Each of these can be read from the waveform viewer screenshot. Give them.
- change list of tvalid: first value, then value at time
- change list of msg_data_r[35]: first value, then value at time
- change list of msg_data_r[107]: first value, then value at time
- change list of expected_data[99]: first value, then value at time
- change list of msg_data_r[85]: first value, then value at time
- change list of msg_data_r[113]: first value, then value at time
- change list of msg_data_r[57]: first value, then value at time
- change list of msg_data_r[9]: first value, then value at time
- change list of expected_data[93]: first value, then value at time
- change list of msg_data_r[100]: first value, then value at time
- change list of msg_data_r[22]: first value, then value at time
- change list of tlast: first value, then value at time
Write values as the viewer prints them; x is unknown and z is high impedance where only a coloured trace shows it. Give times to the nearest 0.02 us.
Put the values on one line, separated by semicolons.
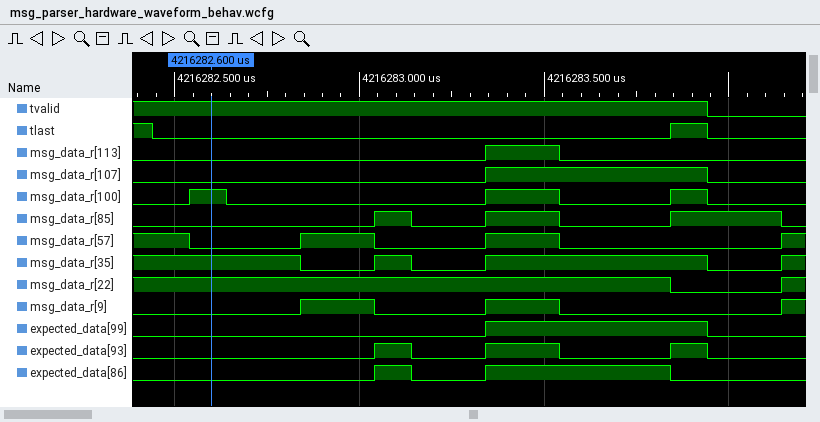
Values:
1, 0 at 4216283.94 us; 1, 0 at 4216282.84 us, 1 at 4216283.04 us, 0 at 4216283.14 us, 1 at 4216283.34 us, 0 at 4216283.94 us, 1 at 4216284.14 us; 0, 1 at 4216283.34 us, 0 at 4216283.94 us; 0, 1 at 4216283.34 us, 0 at 4216283.94 us; 0, 1 at 4216283.04 us, 0 at 4216283.14 us, 1 at 4216283.34 us, 0 at 4216283.54 us, 1 at 4216283.84 us, 0 at 4216284.14 us; 0, 1 at 4216283.34 us, 0 at 4216283.54 us; 1, 0 at 4216282.54 us, 1 at 4216282.84 us, 0 at 4216283.04 us, 1 at 4216283.34 us, 0 at 4216283.54 us, 1 at 4216284.14 us; 0, 1 at 4216282.84 us, 0 at 4216283.04 us, 1 at 4216283.34 us, 0 at 4216283.54 us, 1 at 4216284.14 us; 0, 1 at 4216283.04 us, 0 at 4216283.14 us, 1 at 4216283.34 us, 0 at 4216283.54 us, 1 at 4216283.84 us, 0 at 4216283.94 us; 0, 1 at 4216282.54 us, 0 at 4216282.64 us, 1 at 4216283.34 us, 0 at 4216283.54 us, 1 at 4216283.84 us, 0 at 4216283.94 us; 1, 0 at 4216283.84 us, 1 at 4216284.14 us; 1, 0 at 4216282.44 us, 1 at 4216283.84 us, 0 at 4216283.94 us
